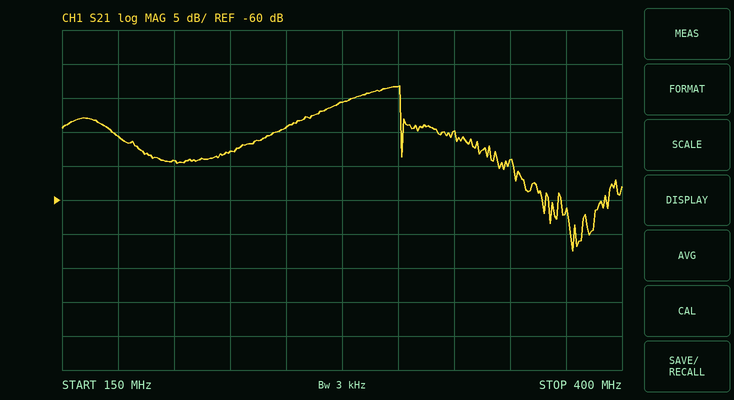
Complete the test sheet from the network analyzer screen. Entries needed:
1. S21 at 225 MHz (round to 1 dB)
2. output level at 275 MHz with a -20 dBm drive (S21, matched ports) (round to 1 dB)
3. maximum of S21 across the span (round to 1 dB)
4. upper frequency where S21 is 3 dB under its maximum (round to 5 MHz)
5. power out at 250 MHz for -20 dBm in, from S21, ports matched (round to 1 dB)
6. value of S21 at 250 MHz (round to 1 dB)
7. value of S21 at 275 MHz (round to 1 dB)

-53 dB
-66 dBm
-43 dB
300 MHz
-69 dBm
-49 dB
-46 dB
